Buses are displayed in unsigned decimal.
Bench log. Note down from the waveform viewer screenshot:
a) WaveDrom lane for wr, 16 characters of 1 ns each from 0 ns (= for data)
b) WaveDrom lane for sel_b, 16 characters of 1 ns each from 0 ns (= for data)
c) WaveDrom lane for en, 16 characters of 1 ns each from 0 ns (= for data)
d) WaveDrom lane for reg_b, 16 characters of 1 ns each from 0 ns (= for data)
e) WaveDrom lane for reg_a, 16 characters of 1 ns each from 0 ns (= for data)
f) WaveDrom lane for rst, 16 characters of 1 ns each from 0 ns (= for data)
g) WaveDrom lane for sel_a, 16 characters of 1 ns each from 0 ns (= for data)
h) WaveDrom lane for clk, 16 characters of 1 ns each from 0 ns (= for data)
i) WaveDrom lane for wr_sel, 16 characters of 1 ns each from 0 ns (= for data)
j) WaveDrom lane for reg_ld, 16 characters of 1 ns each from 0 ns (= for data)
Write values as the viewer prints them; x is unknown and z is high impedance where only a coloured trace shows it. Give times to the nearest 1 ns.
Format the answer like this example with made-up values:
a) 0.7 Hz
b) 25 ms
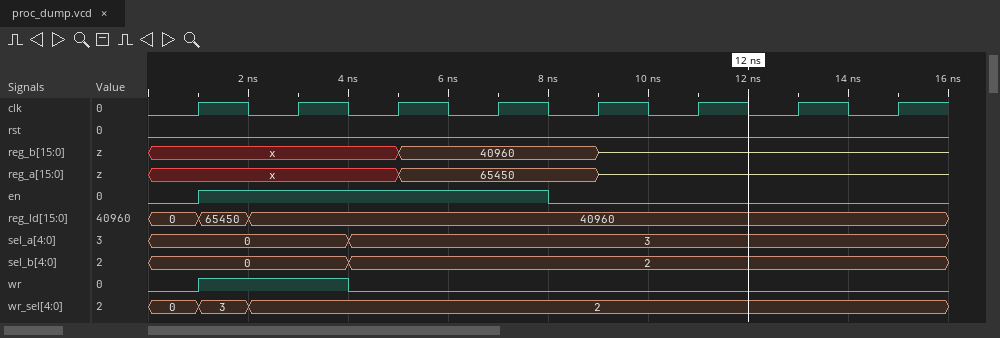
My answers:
a) {name: 'wr', wave: '01..0...........'}
b) {name: 'sel_b', wave: '=...=...........', data: '0 2'}
c) {name: 'en', wave: '01......0.......'}
d) {name: 'reg_b', wave: 'x....=...z......', data: '40960'}
e) {name: 'reg_a', wave: 'x....=...z......', data: '65450'}
f) {name: 'rst', wave: '0...............'}
g) {name: 'sel_a', wave: '=...=...........', data: '0 3'}
h) {name: 'clk', wave: '0101010101010101'}
i) {name: 'wr_sel', wave: '===.............', data: '0 3 2'}
j) {name: 'reg_ld', wave: '===.............', data: '0 65450 40960'}
